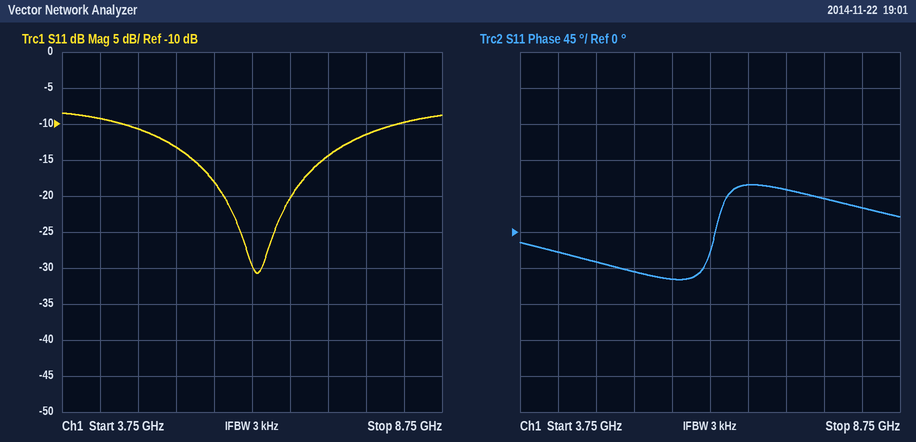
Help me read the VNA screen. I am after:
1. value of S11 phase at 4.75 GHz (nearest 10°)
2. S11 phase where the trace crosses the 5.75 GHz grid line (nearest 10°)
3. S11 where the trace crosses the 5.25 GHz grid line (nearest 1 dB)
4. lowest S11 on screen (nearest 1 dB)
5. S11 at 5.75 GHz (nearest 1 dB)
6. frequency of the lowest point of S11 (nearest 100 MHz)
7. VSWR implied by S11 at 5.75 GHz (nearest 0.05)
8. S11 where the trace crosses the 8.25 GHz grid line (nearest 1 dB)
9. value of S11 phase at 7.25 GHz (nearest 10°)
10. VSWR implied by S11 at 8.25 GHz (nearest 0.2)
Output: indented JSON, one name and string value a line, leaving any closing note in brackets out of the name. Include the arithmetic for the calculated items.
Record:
{
  "value of S11 phase at 4.75 GHz": "-40°",
  "S11 phase where the trace crosses the 5.75 GHz grid line": "-60°",
  "S11 where the trace crosses the 5.25 GHz grid line": "-13 dB",
  "lowest S11 on screen": "-31 dB",
  "S11 at 5.75 GHz": "-18 dB",
  "frequency of the lowest point of S11": "6.3 GHz",
  "VSWR implied by S11 at 5.75 GHz": "|Γ| = 10^(-18/20) = 0.1259; VSWR = (1 + 0.1259)/(1 − 0.1259) ≈ 1.29, so 1.30 to the nearest 0.05",
  "S11 where the trace crosses the 8.25 GHz grid line": "-10 dB",
  "value of S11 phase at 7.25 GHz": "50°",
  "VSWR implied by S11 at 8.25 GHz": "|Γ| = 10^(-10/20) = 0.3162; VSWR = (1 + 0.3162)/(1 − 0.3162) ≈ 1.92, so 2.0 to the nearest 0.2"
}
